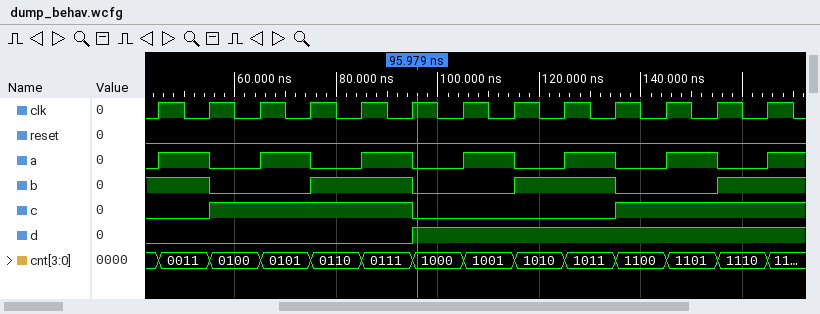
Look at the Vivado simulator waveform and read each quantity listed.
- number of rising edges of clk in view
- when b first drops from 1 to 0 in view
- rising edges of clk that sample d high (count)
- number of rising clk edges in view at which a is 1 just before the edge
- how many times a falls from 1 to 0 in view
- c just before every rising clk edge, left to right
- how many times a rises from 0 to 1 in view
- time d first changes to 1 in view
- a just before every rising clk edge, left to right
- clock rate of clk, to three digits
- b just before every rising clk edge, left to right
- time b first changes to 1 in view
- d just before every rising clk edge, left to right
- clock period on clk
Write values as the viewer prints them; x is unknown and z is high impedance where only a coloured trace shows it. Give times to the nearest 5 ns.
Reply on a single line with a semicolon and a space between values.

13; 55 ns; 7; 6; 6; 0 0 1 1 1 1 0 0 0 0 1 1 1; 7; 95 ns; 0 1 0 1 0 1 0 1 0 1 0 1 0; 100 MHz; 1 1 0 0 1 1 0 0 1 1 0 0 1; 75 ns; 0 0 0 0 0 0 1 1 1 1 1 1 1; 10 ns
